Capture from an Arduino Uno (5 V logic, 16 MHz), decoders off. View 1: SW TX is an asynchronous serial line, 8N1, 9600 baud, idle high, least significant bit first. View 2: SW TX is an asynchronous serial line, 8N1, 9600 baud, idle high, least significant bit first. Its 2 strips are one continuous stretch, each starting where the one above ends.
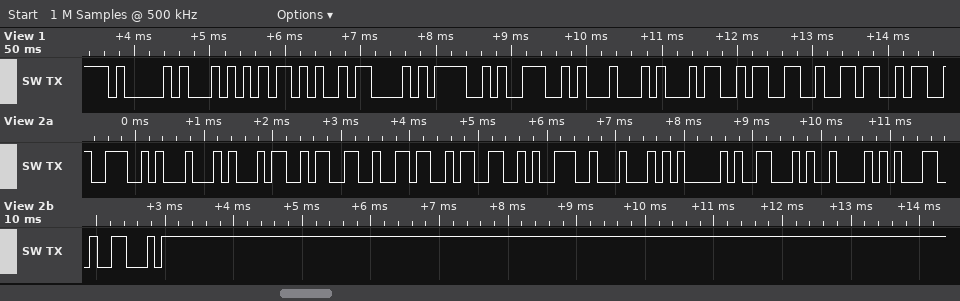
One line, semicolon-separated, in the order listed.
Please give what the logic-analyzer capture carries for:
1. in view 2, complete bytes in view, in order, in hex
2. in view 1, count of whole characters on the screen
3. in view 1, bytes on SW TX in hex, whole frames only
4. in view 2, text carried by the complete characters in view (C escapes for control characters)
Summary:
4E 44 34 33 36 33 39 44 41 46 42 31 46; 10; 41 54 2B 43 4F 4E 44 34 33 36; "ND43639DAFB1F"
